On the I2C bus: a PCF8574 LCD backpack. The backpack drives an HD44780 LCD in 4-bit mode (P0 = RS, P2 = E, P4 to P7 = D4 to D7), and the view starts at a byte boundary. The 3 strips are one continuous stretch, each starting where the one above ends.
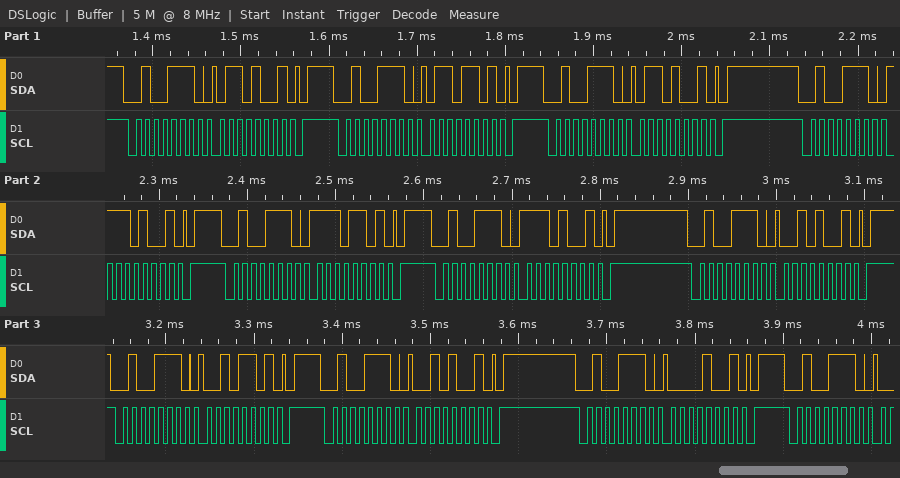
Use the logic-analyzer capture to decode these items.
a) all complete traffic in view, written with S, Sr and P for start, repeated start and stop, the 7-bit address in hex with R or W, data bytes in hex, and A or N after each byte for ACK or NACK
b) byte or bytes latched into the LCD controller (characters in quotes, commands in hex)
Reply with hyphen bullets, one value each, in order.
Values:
- S 27W A 69 A P S 27W A 6D A P S 27W A 69 A P S 27W A E9 A P S 27W A ED A P S 27W A E9 A P S 27W A 29 A P S 27W A 2D A P S 27W A 29 A P S 27W A 09 A P S 27W A
- 'n'
